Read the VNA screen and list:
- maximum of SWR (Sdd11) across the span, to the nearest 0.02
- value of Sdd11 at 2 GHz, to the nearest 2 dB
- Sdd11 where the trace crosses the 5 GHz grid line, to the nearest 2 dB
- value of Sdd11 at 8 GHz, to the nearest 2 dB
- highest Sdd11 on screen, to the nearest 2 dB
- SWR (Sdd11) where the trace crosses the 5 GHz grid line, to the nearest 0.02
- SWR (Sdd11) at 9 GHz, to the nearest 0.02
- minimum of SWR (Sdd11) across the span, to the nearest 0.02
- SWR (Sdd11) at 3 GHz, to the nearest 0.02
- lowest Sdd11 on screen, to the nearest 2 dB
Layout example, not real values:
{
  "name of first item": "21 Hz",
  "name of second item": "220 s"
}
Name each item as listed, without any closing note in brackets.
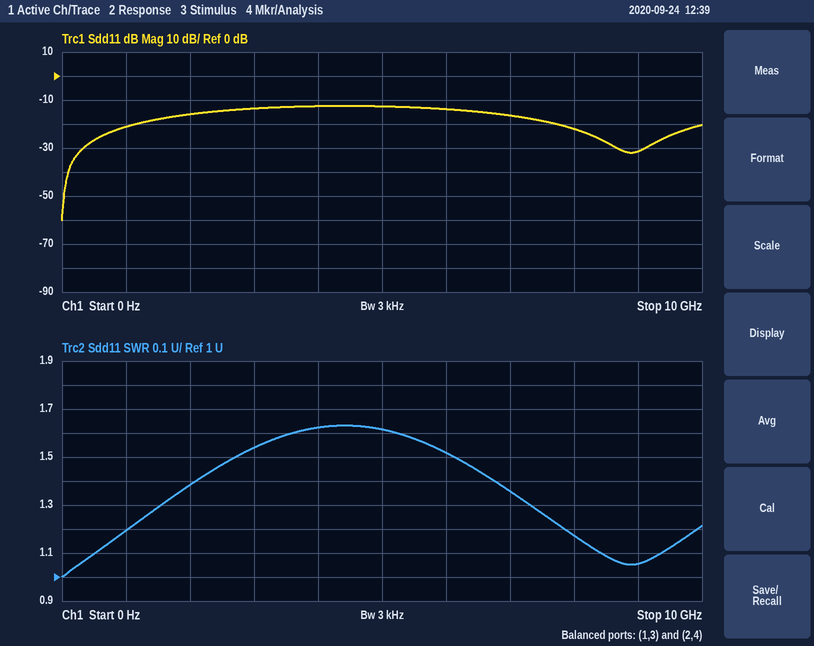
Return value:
{
  "maximum of SWR (Sdd11) across the span, to the nearest 0.02": "1.64",
  "value of Sdd11 at 2 GHz, to the nearest 2 dB": "-16 dB",
  "Sdd11 where the trace crosses the 5 GHz grid line, to the nearest 2 dB": "-12 dB",
  "value of Sdd11 at 8 GHz, to the nearest 2 dB": "-22 dB",
  "highest Sdd11 on screen, to the nearest 2 dB": "-12 dB",
  "SWR (Sdd11) where the trace crosses the 5 GHz grid line, to the nearest 0.02": "1.62",
  "SWR (Sdd11) at 9 GHz, to the nearest 0.02": "1.06",
  "minimum of SWR (Sdd11) across the span, to the nearest 0.02": "1.00",
  "SWR (Sdd11) at 3 GHz, to the nearest 0.02": "1.54",
  "lowest Sdd11 on screen, to the nearest 2 dB": "-60 dB"
}
